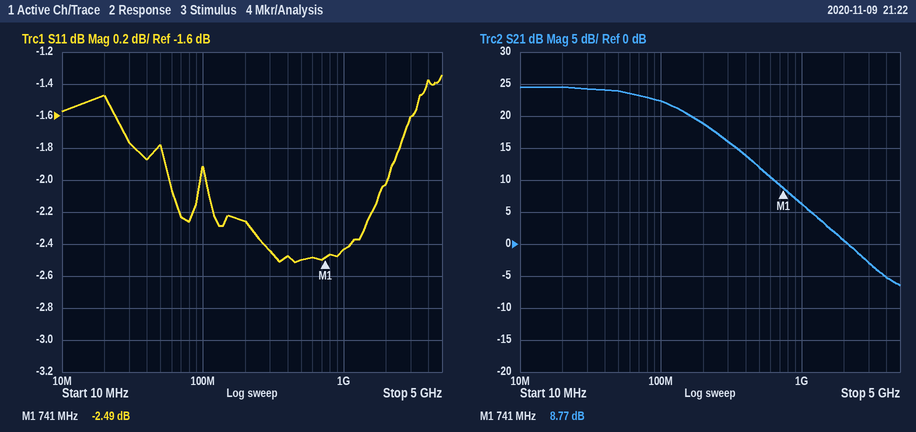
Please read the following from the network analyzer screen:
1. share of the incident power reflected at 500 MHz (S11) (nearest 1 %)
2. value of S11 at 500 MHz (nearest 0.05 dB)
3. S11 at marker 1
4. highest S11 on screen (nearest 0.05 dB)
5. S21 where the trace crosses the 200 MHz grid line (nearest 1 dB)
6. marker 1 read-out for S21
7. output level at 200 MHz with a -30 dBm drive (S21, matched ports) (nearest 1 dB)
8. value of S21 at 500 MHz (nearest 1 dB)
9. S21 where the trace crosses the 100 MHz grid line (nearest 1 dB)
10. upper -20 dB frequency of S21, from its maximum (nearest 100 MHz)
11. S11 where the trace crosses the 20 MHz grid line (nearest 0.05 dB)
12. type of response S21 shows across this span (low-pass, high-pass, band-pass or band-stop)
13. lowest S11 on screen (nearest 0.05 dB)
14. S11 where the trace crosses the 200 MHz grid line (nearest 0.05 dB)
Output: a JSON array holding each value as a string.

["56 %", "-2.50 dB", "-2.49 dB", "-1.35 dB", "19 dB", "8.77 dB", "-11 dBm", "12 dB", "22 dB", "1.2 GHz", "-1.45 dB", "low-pass", "-2.50 dB", "-2.25 dB"]
